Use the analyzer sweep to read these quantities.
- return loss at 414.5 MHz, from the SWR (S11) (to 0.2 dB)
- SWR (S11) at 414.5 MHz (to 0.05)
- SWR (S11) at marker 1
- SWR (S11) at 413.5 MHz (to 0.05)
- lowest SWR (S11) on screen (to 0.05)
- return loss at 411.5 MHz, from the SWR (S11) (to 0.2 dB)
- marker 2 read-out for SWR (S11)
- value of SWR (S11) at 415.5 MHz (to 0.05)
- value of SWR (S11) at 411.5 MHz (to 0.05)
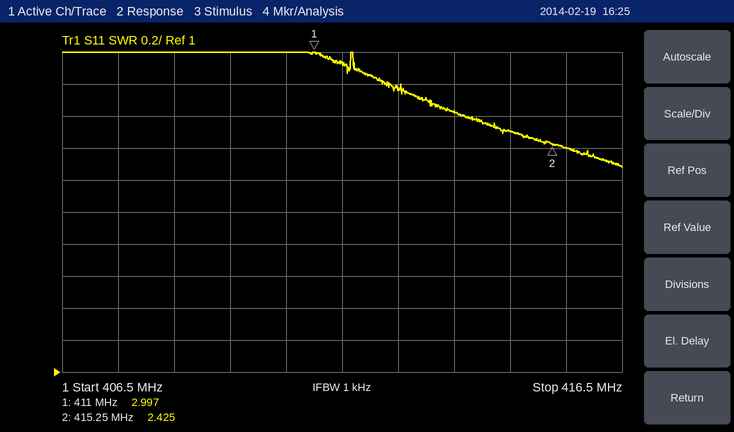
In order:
7.4 dB
2.50
2.997
2.65
2.30
6.2 dB
2.425
2.40
2.95
